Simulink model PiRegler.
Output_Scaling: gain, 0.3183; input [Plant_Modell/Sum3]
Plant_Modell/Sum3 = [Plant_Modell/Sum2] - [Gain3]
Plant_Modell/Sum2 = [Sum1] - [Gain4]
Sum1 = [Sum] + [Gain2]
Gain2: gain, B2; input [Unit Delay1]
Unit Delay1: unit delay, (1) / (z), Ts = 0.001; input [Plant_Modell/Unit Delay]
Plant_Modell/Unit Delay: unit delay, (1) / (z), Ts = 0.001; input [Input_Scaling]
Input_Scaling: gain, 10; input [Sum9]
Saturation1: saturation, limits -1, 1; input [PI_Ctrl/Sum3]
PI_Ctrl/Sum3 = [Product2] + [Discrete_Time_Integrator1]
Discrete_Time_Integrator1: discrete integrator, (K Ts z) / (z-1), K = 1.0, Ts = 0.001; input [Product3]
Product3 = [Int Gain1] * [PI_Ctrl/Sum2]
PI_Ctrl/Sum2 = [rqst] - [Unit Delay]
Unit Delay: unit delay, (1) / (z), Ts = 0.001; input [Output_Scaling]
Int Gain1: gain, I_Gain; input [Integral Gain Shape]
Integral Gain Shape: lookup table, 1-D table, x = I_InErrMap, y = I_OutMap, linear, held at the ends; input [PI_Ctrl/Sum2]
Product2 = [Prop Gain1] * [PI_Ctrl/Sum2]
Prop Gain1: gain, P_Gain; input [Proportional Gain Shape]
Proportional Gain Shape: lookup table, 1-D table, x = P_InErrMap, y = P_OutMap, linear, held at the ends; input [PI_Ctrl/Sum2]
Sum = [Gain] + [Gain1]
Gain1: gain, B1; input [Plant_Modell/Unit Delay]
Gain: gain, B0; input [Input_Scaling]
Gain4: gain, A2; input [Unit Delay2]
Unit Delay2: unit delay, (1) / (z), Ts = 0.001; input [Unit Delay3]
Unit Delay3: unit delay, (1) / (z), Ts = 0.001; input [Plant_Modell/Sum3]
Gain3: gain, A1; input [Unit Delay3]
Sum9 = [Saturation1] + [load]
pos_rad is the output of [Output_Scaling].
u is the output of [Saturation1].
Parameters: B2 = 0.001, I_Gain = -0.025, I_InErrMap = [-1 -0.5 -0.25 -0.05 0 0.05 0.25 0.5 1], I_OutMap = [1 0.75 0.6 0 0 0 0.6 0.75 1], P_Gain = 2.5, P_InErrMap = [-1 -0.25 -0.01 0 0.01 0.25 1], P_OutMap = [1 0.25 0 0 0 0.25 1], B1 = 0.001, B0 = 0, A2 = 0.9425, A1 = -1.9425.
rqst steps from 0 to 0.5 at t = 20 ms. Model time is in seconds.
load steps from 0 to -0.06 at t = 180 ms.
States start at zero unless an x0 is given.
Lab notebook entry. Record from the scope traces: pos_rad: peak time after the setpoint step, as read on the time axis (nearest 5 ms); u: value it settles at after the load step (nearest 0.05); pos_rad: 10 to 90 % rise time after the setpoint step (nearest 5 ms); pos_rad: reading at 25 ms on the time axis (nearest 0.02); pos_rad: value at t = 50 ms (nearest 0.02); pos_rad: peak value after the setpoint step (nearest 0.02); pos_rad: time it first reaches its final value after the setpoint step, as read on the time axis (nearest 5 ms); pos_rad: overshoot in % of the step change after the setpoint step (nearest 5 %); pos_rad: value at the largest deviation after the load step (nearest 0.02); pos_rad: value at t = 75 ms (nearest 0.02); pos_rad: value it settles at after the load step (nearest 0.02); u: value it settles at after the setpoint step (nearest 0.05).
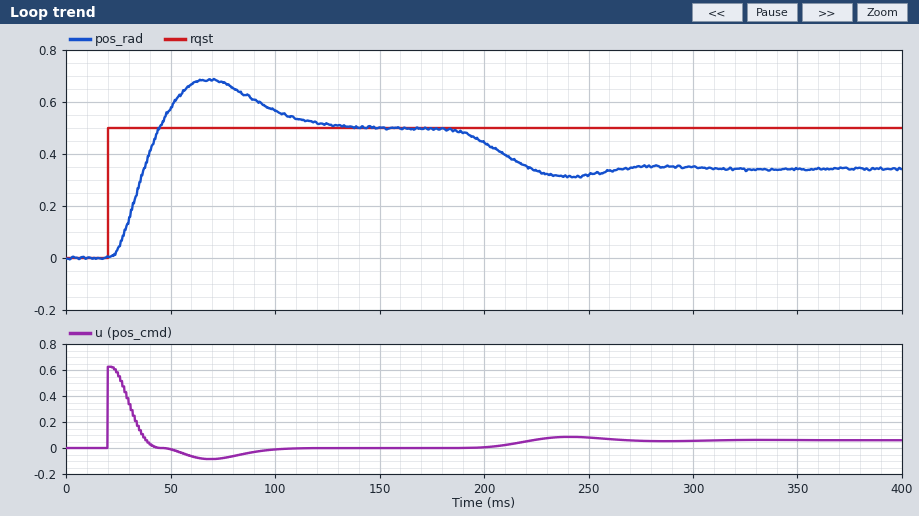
70 ms
0.05
15 ms
0.04
0.58
0.68
45 ms
40 %
0.32
0.68
0.34
0.00
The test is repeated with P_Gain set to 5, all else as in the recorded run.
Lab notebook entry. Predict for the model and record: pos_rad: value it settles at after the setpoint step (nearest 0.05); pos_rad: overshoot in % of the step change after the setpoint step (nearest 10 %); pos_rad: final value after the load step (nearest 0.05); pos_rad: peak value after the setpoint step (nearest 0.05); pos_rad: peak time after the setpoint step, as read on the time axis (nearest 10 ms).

0.50
60 %
0.40
0.80
50 ms
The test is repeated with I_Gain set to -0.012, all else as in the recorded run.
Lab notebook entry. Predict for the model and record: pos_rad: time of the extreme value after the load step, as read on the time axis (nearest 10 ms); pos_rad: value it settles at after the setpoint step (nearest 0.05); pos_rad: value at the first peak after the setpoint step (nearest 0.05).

240 ms
0.50
0.70
